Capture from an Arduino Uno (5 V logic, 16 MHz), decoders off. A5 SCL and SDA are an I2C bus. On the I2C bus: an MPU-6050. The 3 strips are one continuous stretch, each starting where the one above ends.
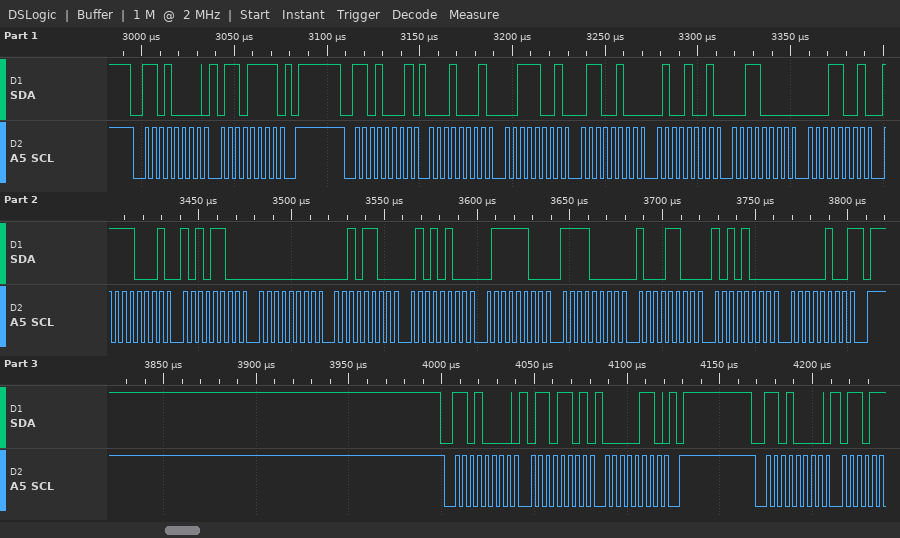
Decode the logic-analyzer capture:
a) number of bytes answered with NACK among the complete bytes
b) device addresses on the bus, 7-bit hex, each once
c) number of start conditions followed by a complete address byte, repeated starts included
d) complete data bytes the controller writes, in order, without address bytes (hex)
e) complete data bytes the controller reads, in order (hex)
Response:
1
0x68
4
6F 6D 06
11 39 64 49 30 19 F1 AC 00 2C 54 7C F0 8C A8 04
